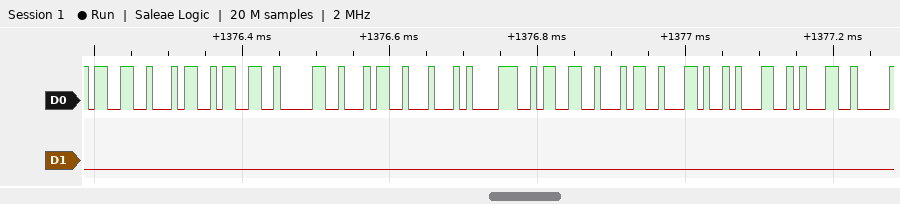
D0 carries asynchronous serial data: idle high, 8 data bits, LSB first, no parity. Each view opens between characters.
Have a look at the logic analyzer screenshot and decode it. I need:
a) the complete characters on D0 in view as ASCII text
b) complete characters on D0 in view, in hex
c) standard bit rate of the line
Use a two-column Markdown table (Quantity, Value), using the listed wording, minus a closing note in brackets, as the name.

| Quantity | Value |
|---|---|
| the complete characters on D0 in view as ASCII text | "34304D834,11" |
| complete characters on D0 in view, in hex | 33, 34, 33, 30, 34, 44, 38, 33, 34, 2C, 31, 31 |
| standard bit rate of the line | 115200 baud |
